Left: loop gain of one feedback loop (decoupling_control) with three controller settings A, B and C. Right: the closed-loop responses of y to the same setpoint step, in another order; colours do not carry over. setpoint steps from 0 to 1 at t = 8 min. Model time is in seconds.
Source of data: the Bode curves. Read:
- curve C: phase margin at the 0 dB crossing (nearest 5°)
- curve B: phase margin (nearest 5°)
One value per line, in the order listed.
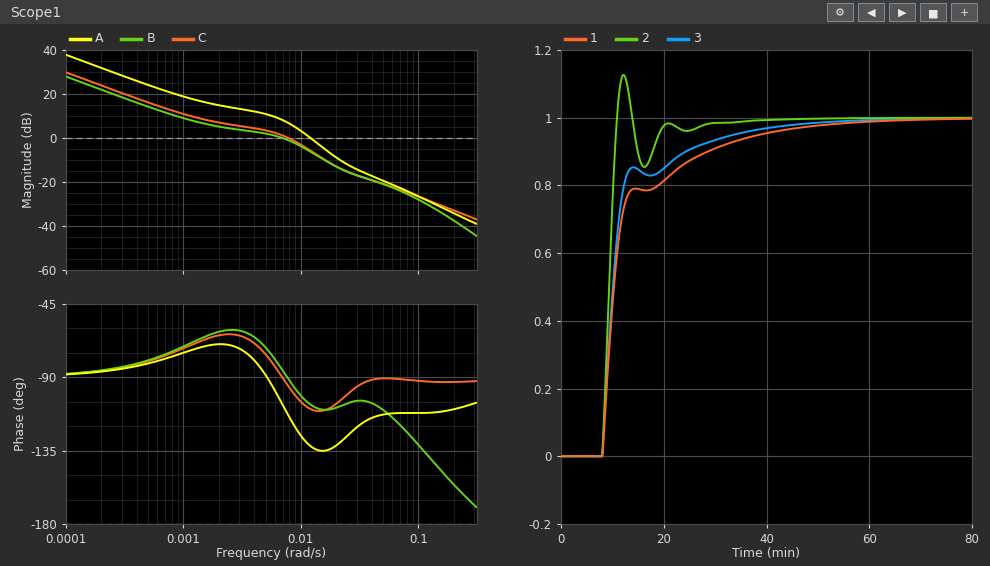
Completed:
85°
95°
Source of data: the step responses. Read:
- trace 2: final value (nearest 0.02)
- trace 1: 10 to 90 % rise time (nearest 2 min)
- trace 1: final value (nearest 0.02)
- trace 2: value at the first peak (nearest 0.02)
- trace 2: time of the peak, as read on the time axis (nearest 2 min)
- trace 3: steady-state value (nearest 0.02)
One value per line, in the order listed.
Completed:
1.00
20 min
1.00
1.12
12 min
1.00
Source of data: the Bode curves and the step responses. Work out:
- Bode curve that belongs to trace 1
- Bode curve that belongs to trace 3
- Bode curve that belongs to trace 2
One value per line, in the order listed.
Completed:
B
C
A
